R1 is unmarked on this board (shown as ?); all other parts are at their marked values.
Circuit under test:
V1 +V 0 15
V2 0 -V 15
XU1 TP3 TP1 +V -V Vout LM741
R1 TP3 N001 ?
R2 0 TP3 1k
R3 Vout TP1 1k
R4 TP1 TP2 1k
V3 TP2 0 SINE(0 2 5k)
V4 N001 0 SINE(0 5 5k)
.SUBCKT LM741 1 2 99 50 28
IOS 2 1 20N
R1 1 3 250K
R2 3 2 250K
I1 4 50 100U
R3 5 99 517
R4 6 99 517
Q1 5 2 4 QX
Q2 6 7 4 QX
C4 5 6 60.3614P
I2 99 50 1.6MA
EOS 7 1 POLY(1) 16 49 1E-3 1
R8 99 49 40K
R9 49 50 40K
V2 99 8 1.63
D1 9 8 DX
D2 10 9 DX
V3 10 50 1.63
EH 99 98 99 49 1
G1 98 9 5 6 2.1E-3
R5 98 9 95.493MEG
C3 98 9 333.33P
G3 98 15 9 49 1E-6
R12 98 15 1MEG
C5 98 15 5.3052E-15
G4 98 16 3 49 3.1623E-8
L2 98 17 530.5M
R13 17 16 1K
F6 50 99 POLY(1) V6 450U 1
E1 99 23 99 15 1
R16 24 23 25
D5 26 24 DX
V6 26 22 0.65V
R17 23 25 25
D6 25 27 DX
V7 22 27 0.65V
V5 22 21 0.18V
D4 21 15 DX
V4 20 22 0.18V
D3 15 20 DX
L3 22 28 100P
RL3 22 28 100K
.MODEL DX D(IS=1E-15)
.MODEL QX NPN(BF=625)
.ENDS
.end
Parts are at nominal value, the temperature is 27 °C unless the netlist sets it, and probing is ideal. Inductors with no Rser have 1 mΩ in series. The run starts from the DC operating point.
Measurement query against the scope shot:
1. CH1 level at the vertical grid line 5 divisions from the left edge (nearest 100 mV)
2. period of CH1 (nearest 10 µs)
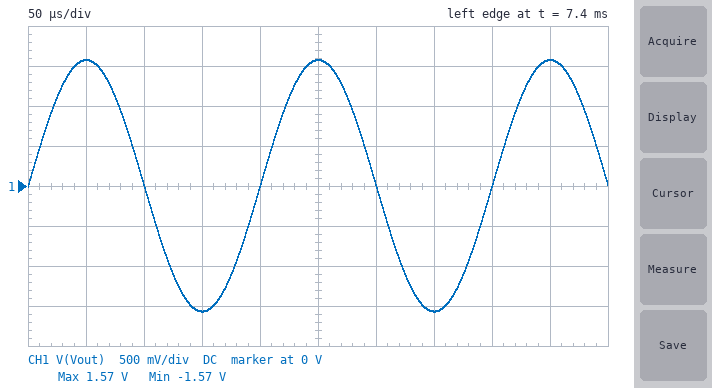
1.6 V
200 µs
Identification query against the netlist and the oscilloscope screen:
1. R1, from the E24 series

1.8 kΩ
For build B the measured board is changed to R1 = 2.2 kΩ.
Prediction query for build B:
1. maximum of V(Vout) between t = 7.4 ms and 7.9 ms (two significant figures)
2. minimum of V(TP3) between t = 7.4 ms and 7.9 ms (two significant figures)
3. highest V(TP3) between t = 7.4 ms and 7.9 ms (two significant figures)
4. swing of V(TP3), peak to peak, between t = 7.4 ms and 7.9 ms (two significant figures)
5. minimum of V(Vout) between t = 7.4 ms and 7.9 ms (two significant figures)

1.1 V
-1.6 V
1.6 V
3.1 V
-1.1 V
